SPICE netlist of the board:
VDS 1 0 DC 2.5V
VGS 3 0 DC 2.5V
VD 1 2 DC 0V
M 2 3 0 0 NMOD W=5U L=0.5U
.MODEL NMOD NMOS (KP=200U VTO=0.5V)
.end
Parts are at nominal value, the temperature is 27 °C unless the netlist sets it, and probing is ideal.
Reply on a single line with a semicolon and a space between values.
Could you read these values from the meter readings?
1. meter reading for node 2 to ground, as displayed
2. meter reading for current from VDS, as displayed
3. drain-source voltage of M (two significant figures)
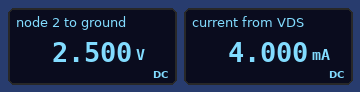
2.500 V; 4.000 mA; 2.5 V
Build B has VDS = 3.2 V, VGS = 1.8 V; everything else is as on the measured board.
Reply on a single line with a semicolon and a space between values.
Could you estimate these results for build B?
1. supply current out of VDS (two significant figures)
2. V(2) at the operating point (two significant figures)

1.7 mA; 3.2 V
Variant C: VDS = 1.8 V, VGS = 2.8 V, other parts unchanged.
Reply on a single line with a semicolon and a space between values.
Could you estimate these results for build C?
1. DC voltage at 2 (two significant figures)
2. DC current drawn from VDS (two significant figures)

1.8 V; 5.0 mA
